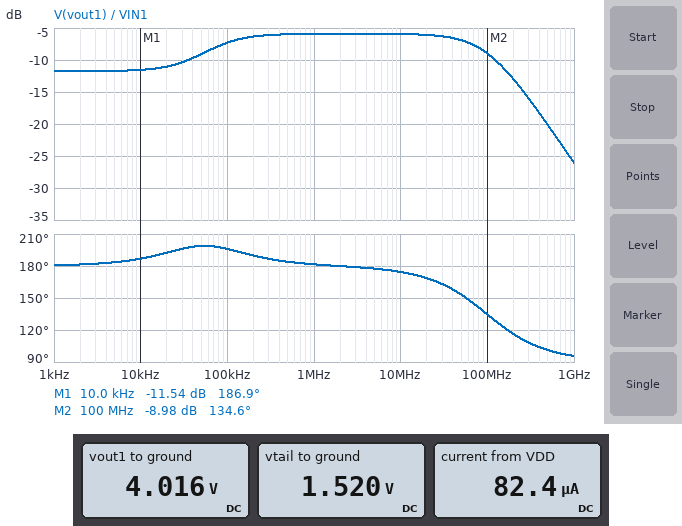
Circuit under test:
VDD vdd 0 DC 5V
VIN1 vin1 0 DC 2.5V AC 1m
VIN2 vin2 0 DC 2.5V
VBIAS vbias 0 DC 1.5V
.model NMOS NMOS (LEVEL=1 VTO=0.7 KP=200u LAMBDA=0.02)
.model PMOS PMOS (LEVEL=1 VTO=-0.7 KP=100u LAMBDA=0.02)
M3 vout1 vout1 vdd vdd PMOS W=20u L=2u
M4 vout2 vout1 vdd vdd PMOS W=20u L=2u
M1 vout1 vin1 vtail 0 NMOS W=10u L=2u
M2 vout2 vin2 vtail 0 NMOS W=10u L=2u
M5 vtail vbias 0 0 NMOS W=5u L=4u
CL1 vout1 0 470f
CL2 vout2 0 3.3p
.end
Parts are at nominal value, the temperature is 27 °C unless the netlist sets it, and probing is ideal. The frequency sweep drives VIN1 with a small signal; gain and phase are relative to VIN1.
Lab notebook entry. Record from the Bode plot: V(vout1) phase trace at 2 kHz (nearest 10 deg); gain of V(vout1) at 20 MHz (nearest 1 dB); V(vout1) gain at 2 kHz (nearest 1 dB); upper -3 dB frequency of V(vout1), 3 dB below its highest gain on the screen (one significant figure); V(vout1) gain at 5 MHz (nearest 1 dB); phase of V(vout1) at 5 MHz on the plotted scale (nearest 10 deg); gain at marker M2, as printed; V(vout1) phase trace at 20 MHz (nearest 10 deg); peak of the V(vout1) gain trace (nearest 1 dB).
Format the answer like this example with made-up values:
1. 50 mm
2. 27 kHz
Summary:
1. 180 deg
2. -6 dB
3. -12 dB
4. 100 MHz
5. -6 dB
6. 180 deg
7. -8.98 dB
8. 170 deg
9. -6 dB
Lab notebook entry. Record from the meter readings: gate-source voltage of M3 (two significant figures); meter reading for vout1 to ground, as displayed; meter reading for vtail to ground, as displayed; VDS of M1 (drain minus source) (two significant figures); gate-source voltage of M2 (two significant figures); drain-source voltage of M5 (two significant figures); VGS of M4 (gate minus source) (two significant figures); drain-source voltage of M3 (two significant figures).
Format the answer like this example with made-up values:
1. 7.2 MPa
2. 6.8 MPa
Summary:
1. -980 mV
2. 4.016 V
3. 1.520 V
4. 2.5 V
5. 980 mV
6. 1.5 V
7. -980 mV
8. -980 mV
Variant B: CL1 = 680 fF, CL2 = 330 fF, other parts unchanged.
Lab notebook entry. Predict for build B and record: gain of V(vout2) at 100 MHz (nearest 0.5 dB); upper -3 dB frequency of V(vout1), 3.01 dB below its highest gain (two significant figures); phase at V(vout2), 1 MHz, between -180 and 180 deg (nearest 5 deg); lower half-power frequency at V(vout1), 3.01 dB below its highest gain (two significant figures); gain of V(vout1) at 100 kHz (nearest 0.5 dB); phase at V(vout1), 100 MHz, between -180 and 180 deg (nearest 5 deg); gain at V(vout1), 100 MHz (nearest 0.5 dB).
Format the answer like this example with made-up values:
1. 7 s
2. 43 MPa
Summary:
1. 0 dB
2. 69 MHz
3. -55 deg
4. 520 kHz
5. -11.5 dB
6. 125 deg
7. -11.0 dB
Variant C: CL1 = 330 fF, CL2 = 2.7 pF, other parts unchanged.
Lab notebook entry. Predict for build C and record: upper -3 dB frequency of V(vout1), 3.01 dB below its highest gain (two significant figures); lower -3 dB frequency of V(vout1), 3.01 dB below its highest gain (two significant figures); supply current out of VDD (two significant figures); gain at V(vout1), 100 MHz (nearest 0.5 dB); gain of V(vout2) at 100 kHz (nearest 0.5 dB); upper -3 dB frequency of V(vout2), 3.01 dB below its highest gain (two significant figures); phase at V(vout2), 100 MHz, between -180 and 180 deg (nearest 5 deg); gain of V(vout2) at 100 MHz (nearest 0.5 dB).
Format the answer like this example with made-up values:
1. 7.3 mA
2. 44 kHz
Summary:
1. 140 MHz
2. 65 kHz
3. 82 µA
4. -7.5 dB
5. 42.0 dB
6. 94 kHz
7. -105 deg
8. -16.5 dB
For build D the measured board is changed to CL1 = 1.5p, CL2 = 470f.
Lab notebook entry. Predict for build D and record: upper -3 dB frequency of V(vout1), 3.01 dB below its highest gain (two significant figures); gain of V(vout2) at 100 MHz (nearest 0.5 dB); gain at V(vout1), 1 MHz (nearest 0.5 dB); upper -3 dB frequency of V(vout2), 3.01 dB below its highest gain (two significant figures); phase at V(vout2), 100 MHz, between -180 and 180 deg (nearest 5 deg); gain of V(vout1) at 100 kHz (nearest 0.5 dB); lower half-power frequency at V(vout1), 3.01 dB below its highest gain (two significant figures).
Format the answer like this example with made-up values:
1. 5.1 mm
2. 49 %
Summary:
1. 32 MHz
2. -5.0 dB
3. -6.5 dB
4. 540 kHz
5. -105 deg
6. -11.5 dB
7. 360 kHz
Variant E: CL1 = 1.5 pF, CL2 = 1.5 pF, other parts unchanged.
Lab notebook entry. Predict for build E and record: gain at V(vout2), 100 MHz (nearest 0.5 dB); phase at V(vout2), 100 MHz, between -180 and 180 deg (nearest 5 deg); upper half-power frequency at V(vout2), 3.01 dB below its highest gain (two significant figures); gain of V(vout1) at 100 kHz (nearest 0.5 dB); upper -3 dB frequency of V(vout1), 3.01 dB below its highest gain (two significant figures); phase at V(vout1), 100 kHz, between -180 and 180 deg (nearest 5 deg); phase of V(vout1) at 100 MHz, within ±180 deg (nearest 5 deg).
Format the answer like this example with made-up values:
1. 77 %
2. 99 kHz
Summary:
1. -15.0 dB
2. -105 deg
3. 170 kHz
4. -9.5 dB
5. 31 MHz
6. -160 deg
7. 105 deg
